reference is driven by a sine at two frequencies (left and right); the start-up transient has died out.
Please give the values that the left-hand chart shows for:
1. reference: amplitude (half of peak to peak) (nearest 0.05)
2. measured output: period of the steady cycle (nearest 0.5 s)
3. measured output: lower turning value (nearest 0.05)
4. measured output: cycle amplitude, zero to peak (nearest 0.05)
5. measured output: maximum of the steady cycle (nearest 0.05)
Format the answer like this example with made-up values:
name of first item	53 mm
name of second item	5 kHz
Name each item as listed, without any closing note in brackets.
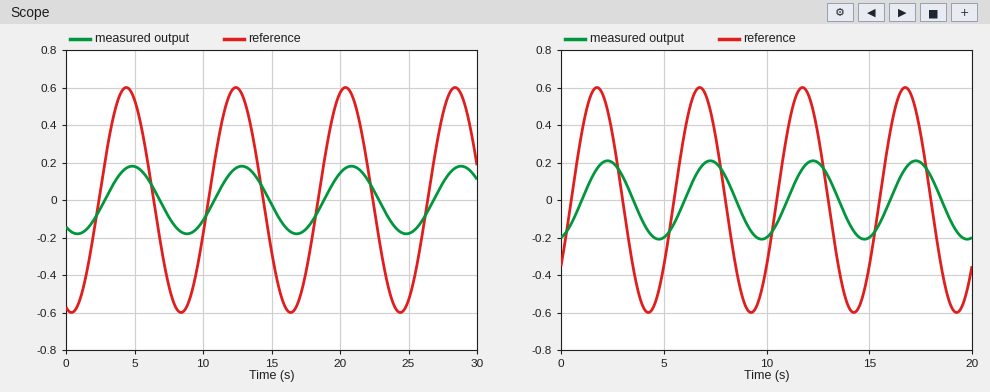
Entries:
reference: amplitude (half of peak to peak)	0.60
measured output: period of the steady cycle	8.0 s
measured output: lower turning value	-0.20
measured output: cycle amplitude, zero to peak	0.20
measured output: maximum of the steady cycle	0.20
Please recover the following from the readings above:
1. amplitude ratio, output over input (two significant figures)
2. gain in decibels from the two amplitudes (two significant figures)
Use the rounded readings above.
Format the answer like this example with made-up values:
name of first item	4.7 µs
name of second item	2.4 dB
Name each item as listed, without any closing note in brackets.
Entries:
amplitude ratio, output over input	0.33
gain in decibels from the two amplitudes	-9.5 dB
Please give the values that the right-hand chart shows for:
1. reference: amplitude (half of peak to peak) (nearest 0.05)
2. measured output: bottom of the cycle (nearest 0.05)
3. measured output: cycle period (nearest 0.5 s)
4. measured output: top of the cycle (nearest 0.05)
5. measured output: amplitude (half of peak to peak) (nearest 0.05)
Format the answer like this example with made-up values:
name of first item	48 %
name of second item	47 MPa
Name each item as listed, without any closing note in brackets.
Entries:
reference: amplitude (half of peak to peak)	0.60
measured output: bottom of the cycle	-0.20
measured output: cycle period	5.0 s
measured output: top of the cycle	0.20
measured output: amplitude (half of peak to peak)	0.20
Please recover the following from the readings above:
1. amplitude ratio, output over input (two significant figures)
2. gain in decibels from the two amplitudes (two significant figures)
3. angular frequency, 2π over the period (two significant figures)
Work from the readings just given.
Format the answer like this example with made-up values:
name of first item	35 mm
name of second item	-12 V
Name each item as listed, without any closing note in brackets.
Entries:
amplitude ratio, output over input	0.33
gain in decibels from the two amplitudes	-9.5 dB
angular frequency, 2π over the period	1.3 rad/s
